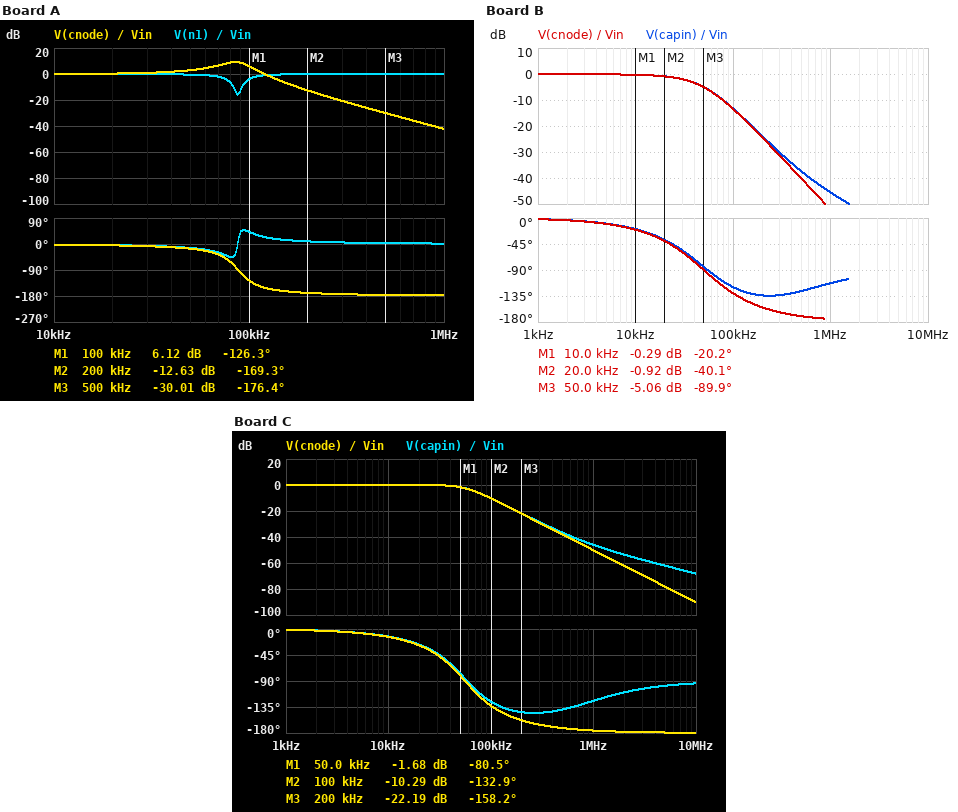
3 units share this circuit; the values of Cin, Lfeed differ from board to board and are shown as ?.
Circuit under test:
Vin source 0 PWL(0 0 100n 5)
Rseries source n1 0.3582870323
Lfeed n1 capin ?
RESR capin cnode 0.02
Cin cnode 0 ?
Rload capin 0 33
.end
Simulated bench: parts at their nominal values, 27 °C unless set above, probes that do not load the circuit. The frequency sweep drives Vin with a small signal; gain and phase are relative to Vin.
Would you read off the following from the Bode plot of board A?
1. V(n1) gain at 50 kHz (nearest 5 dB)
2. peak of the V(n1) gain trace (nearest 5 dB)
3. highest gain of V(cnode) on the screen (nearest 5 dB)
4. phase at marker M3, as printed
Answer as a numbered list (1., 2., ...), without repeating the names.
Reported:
1. 0 dB
2. 0 dB
3. 10 dB
4. -176.4 deg
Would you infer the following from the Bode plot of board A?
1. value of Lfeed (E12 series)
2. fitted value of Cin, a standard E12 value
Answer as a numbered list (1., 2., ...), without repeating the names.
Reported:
1. 2.2 µH
2. 1.5 µF
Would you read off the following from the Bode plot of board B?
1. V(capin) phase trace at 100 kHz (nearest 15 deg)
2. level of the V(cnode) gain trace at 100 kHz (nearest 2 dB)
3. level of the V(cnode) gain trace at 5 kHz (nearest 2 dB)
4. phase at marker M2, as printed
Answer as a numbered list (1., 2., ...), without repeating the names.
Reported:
1. -120 deg
2. -14 dB
3. 0 dB
4. -40.1 deg
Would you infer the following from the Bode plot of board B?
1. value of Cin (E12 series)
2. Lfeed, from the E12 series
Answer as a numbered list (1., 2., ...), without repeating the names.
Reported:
1. 15 µF
2. 680 nH
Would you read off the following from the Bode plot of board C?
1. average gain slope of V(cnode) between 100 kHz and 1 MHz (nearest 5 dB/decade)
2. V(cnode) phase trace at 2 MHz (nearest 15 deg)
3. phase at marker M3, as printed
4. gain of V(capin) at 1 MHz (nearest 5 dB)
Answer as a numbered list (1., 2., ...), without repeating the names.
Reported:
1. -40 dB/decade
2. -180 deg
3. -158.2 deg
4. -45 dB
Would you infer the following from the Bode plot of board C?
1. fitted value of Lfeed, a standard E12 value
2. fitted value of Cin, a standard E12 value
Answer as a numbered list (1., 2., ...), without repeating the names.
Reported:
1. 820 nH
2. 10 µF
